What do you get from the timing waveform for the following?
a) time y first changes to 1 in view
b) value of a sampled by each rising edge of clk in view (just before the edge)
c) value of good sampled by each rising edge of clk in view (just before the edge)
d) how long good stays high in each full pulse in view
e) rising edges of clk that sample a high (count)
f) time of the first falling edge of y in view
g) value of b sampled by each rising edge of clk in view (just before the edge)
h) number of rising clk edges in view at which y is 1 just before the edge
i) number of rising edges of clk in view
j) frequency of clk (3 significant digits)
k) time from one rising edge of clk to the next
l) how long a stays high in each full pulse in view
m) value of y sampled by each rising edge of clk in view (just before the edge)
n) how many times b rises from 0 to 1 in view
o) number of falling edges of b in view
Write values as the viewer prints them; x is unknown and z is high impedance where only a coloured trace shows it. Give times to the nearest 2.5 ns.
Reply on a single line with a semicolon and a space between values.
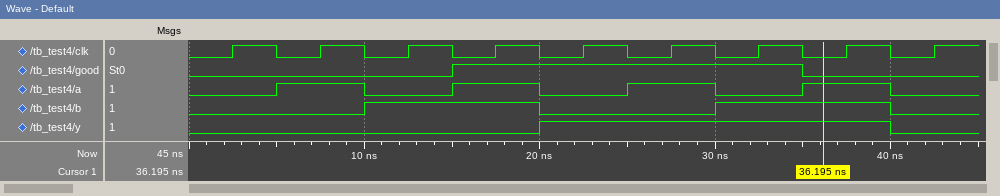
20 ns; 0 1 0 1 0 1 0 1 0; 0 0 0 1 1 1 1 0 0; 20 ns; 4; 40 ns; 0 0 1 1 0 0 1 1 0; 4; 9; 200 MHz; 5 ns; 5 ns, 5 ns, 5 ns, 5 ns; 0 0 0 0 1 1 1 1 0; 2; 2
